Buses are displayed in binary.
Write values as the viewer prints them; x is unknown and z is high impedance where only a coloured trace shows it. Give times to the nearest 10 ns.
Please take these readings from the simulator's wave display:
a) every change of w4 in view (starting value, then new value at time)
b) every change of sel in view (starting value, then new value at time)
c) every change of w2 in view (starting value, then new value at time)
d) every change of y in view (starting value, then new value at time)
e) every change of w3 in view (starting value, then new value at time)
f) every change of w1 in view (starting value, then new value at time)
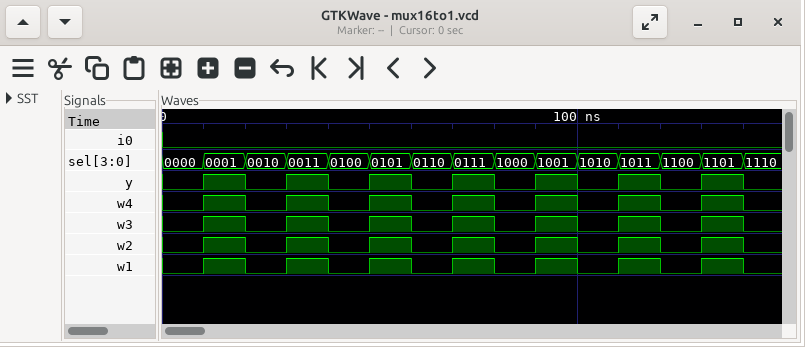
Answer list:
0, 1 at 10 ns, 0 at 20 ns, 1 at 30 ns, 0 at 40 ns, 1 at 50 ns, 0 at 60 ns, 1 at 70 ns, 0 at 80 ns, 1 at 90 ns, 0 at 100 ns, 1 at 110 ns, 0 at 120 ns, 1 at 130 ns, 0 at 140 ns
0000, 0001 at 10 ns, 0010 at 20 ns, 0011 at 30 ns, 0100 at 40 ns, 0101 at 50 ns, 0110 at 60 ns, 0111 at 70 ns, 1000 at 80 ns, 1001 at 90 ns, 1010 at 100 ns, 1011 at 110 ns, 1100 at 120 ns, 1101 at 130 ns, 1110 at 140 ns
0, 1 at 10 ns, 0 at 20 ns, 1 at 30 ns, 0 at 40 ns, 1 at 50 ns, 0 at 60 ns, 1 at 70 ns, 0 at 80 ns, 1 at 90 ns, 0 at 100 ns, 1 at 110 ns, 0 at 120 ns, 1 at 130 ns, 0 at 140 ns
0, 1 at 10 ns, 0 at 20 ns, 1 at 30 ns, 0 at 40 ns, 1 at 50 ns, 0 at 60 ns, 1 at 70 ns, 0 at 80 ns, 1 at 90 ns, 0 at 100 ns, 1 at 110 ns, 0 at 120 ns, 1 at 130 ns, 0 at 140 ns
0, 1 at 10 ns, 0 at 20 ns, 1 at 30 ns, 0 at 40 ns, 1 at 50 ns, 0 at 60 ns, 1 at 70 ns, 0 at 80 ns, 1 at 90 ns, 0 at 100 ns, 1 at 110 ns, 0 at 120 ns, 1 at 130 ns, 0 at 140 ns
0, 1 at 10 ns, 0 at 20 ns, 1 at 30 ns, 0 at 40 ns, 1 at 50 ns, 0 at 60 ns, 1 at 70 ns, 0 at 80 ns, 1 at 90 ns, 0 at 100 ns, 1 at 110 ns, 0 at 120 ns, 1 at 130 ns, 0 at 140 ns
